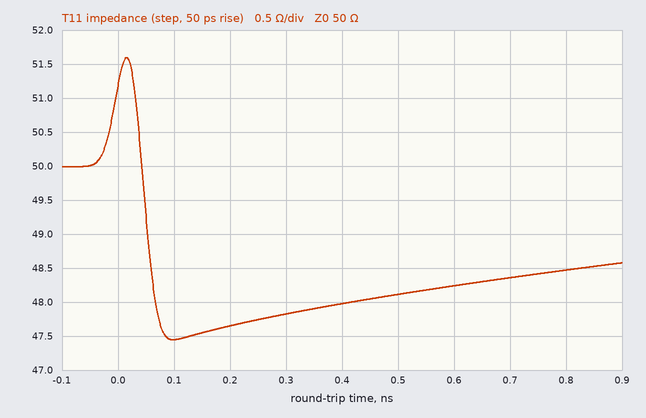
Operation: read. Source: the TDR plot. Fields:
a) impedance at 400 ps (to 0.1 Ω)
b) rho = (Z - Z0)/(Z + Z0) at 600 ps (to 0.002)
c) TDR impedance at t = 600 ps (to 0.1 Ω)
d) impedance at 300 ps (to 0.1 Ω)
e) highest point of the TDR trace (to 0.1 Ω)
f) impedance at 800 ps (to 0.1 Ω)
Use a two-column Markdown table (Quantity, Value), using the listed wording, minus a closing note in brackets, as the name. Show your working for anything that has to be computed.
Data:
| Quantity | Value |
|---|---|
| impedance at 400 ps | 48.0 Ω |
| rho = (Z - Z0)/(Z + Z0) at 600 ps | (48.2 − 50)/(48.2 + 50) ≈ -0.018 |
| TDR impedance at t = 600 ps | 48.2 Ω |
| impedance at 300 ps | 47.8 Ω |
| highest point of the TDR trace | 51.6 Ω |
| impedance at 800 ps | 48.5 Ω |
